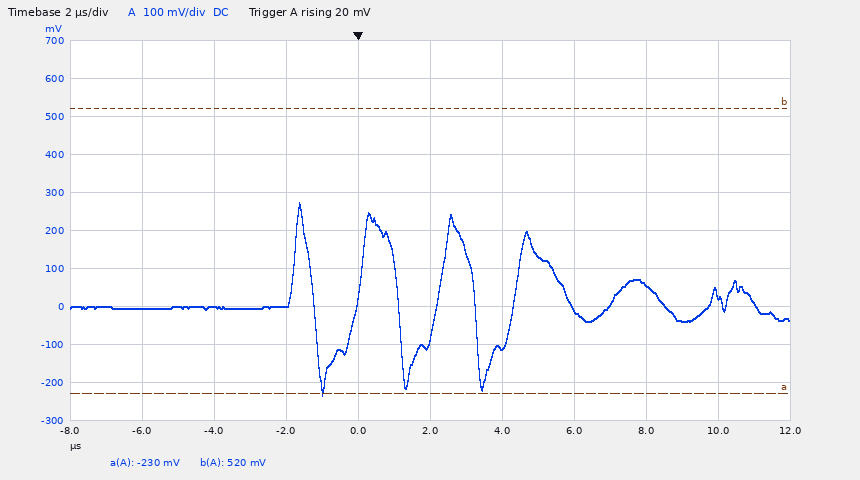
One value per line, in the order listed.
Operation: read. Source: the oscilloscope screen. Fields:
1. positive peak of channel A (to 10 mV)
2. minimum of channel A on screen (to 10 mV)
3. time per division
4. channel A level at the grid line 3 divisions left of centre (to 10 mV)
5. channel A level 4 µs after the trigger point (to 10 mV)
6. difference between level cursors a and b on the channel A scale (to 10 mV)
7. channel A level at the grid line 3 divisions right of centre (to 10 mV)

270 mV
-230 mV
2 µs
0 mV
-110 mV
750 mV
60 mV
